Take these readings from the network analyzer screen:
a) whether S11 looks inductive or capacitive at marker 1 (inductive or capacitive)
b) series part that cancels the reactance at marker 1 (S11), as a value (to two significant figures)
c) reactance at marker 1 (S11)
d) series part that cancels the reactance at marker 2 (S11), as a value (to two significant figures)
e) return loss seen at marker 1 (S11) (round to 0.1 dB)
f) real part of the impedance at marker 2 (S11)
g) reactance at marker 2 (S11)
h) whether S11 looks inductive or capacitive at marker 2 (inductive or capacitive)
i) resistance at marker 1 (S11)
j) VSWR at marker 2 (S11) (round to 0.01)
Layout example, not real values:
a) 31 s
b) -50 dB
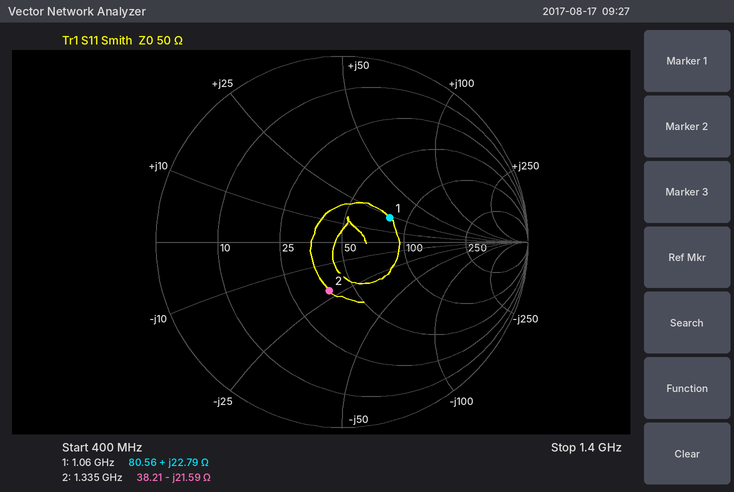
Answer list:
a) inductive
b) 6.6 pF
c) +22.79 Ω
d) 2.6 nH
e) 10.8 dB
f) 38.21 Ω
g) -21.59 Ω
h) capacitive
i) 80.56 Ω
j) 1.74
